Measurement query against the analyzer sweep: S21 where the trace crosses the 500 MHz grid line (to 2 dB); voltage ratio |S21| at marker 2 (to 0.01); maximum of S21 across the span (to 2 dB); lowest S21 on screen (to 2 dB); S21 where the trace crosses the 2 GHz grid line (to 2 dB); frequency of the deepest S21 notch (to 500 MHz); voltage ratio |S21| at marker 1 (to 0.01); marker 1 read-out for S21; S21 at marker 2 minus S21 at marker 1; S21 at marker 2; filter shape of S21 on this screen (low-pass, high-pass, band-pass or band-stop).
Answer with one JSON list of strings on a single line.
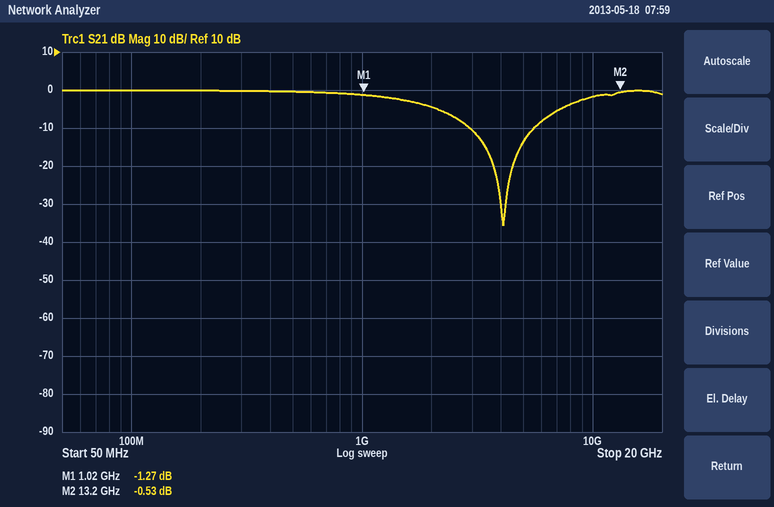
["0 dB", "0.94", "0 dB", "-36 dB", "-4 dB", "4.0 GHz", "0.86", "-1.27 dB", "0.74 dB", "-0.53 dB", "band-stop"]
